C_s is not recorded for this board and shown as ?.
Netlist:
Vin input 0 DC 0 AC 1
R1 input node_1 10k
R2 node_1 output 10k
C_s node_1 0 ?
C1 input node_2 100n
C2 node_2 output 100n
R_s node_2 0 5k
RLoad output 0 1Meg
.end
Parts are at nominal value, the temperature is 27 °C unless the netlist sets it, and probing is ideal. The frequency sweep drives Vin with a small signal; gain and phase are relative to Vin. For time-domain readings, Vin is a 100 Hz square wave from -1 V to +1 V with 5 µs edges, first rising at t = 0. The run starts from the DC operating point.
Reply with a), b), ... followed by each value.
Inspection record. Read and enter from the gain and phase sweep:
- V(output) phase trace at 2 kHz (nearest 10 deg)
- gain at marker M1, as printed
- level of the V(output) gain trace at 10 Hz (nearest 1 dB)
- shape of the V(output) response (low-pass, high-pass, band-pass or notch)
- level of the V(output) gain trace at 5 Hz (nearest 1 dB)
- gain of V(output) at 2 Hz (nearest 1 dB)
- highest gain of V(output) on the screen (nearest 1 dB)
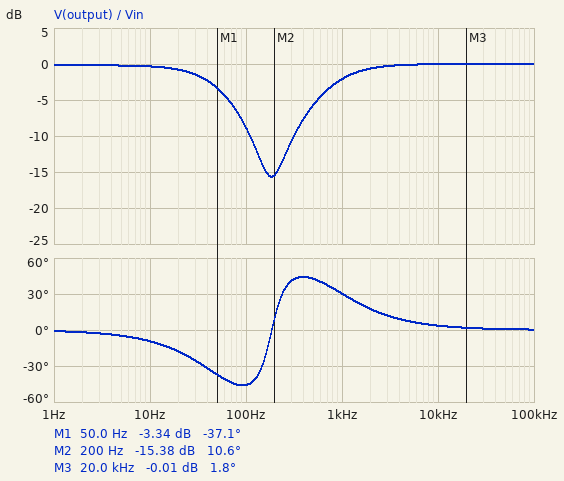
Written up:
a) 20 deg
b) -3.34 dB
c) 0 dB
d) notch
e) 0 dB
f) 0 dB
g) 0 dB
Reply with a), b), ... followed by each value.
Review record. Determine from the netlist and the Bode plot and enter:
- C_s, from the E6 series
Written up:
a) 68 nF
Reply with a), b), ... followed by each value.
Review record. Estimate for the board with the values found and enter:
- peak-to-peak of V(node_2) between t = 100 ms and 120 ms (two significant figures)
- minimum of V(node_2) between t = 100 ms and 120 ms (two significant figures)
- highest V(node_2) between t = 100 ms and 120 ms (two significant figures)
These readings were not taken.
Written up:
a) 3.8 V
b) -1.9 V
c) 1.9 V
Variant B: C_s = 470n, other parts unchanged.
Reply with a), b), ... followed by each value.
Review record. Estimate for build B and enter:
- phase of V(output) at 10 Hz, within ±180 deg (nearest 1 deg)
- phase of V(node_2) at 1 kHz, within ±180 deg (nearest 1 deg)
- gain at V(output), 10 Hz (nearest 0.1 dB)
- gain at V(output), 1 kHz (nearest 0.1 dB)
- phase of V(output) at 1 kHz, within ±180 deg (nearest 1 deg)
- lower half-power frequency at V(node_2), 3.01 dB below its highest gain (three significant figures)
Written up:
a) -23 deg
b) 25 deg
c) -0.8 dB
d) -1.3 dB
e) 34 deg
f) 536 Hz
